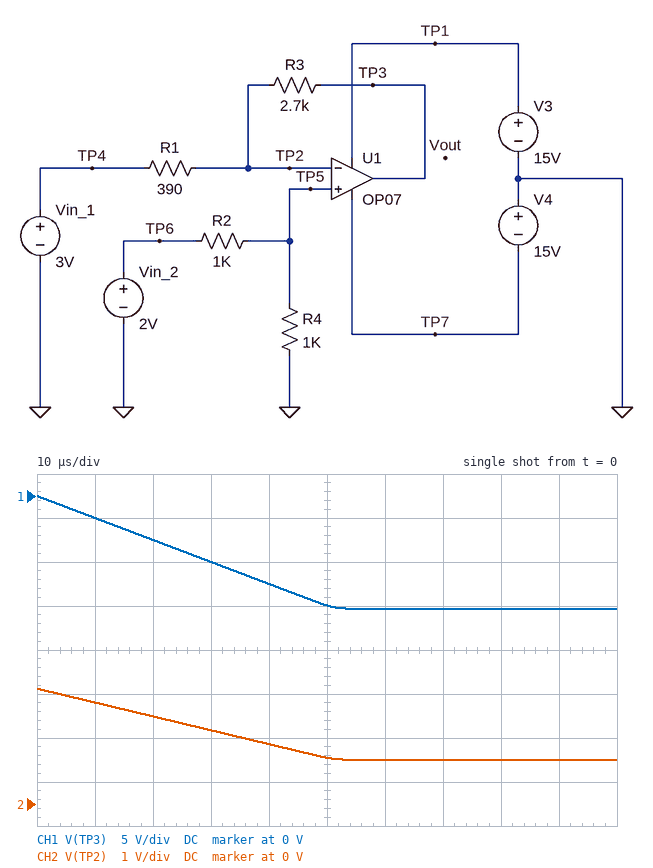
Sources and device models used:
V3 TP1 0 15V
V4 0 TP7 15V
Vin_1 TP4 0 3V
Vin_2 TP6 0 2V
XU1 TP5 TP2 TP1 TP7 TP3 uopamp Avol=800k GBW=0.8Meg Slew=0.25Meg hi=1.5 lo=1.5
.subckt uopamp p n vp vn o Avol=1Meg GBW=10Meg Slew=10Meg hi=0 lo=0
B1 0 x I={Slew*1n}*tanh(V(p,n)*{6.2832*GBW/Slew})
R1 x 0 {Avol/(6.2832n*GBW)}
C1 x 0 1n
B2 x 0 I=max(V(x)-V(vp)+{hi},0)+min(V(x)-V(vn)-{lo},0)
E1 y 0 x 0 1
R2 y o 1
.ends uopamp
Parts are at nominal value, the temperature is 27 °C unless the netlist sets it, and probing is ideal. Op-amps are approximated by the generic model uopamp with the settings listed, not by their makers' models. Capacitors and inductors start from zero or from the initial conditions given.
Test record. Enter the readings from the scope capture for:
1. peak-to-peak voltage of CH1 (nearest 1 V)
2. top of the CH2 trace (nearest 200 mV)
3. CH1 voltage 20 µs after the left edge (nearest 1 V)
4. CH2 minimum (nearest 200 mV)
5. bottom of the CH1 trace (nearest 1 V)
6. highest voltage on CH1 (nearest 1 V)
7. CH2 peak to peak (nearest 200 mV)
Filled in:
13 V
2.6 V
-5 V
1.0 V
-13 V
0 V
1.6 V
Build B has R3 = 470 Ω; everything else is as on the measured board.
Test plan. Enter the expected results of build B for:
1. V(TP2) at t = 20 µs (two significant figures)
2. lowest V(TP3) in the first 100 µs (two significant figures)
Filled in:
1.0 V
-1.4 V
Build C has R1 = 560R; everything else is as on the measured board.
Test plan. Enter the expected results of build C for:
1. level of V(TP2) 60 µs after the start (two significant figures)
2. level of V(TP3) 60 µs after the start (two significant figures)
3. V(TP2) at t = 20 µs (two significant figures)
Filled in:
1.0 V
-8.6 V
1.6 V
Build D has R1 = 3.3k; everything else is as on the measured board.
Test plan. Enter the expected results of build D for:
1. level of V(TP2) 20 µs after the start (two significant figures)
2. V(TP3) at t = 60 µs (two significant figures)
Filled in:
1.0 V
-640 mV
